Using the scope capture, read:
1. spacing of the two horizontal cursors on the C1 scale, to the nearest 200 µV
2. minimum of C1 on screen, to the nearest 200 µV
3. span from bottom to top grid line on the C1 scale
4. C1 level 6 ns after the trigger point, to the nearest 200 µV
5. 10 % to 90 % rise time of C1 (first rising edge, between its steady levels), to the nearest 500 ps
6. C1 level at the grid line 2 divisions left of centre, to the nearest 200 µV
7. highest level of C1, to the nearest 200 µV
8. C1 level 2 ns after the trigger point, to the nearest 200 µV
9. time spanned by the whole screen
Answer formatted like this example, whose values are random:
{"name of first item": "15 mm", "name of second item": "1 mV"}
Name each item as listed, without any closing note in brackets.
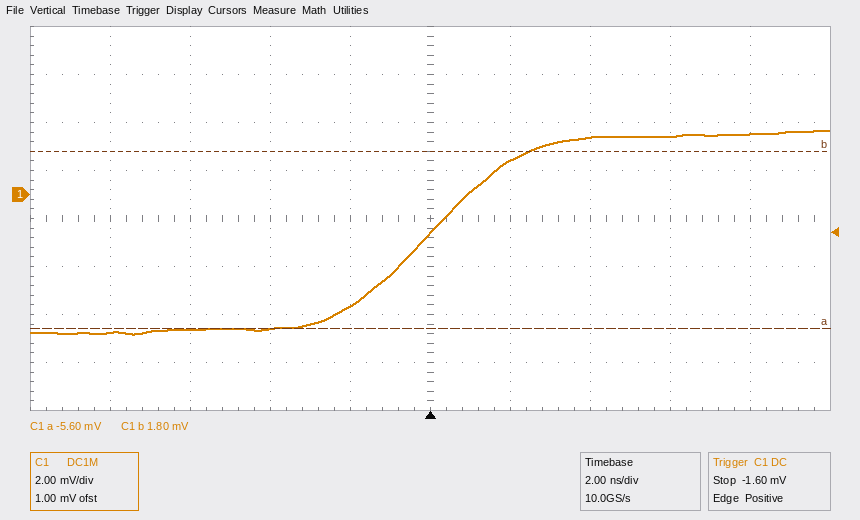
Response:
{"spacing of the two horizontal cursors on the C1 scale, to the nearest 200 µV": "7.4 mV", "minimum of C1 on screen, to the nearest 200 µV": "-5.8 mV", "span from bottom to top grid line on the C1 scale": "16 mV", "C1 level 6 ns after the trigger point, to the nearest 200 µV": "2.4 mV", "10 % to 90 % rise time of C1 (first rising edge, between its steady levels), to the nearest 500 ps": "4.5 ns", "C1 level at the grid line 2 divisions left of centre, to the nearest 200 µV": "-5.6 mV", "highest level of C1, to the nearest 200 µV": "2.6 mV", "C1 level 2 ns after the trigger point, to the nearest 200 µV": "1.4 mV", "time spanned by the whole screen": "20 ns"}
